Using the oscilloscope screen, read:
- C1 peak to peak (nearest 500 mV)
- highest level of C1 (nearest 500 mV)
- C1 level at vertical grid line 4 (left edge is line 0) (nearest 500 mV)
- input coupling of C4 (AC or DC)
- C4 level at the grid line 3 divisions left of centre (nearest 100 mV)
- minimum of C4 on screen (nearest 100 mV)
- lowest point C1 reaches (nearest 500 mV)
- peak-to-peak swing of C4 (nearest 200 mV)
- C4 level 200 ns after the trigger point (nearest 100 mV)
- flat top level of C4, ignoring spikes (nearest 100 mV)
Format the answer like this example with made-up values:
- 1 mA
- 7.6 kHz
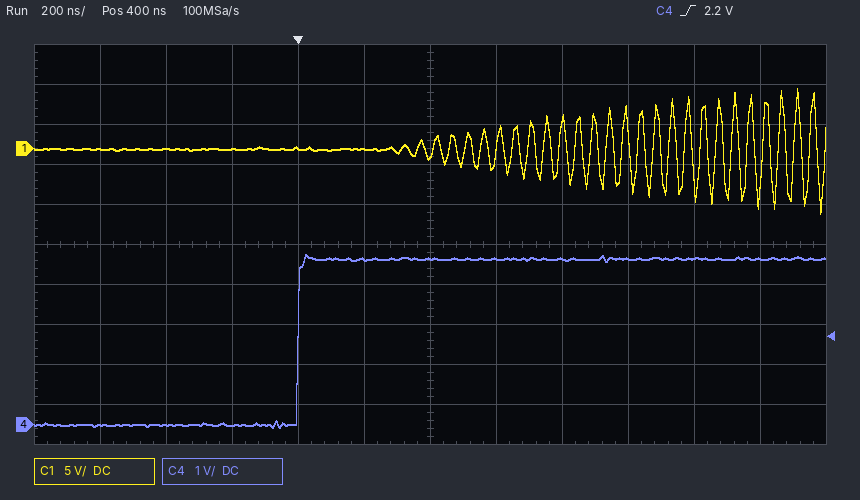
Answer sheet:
- 15.5 V
- 7.5 V
- 0.0 V
- DC
- 0.0 V
- -100 mV
- -8.0 V
- 4.4 V
- 4.1 V
- 4.1 V
